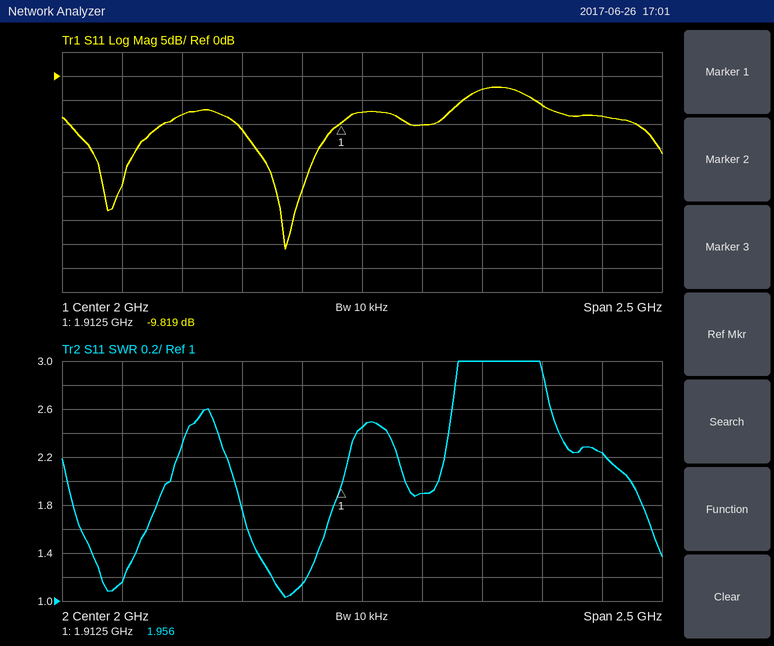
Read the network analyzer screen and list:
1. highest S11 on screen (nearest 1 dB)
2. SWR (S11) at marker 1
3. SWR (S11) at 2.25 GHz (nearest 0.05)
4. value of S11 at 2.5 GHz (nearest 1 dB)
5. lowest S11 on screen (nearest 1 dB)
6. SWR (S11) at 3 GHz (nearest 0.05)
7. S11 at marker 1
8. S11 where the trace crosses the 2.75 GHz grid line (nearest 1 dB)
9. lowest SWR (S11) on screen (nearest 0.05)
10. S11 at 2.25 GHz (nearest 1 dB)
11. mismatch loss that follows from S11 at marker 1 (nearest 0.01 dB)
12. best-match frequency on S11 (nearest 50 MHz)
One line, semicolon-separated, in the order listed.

-2 dB; 1.956; 1.90; -3 dB; -36 dB; 2.25; -9.819 dB; -6 dB; 1.05; -10 dB; 0.48 dB; 1.70 GHz
